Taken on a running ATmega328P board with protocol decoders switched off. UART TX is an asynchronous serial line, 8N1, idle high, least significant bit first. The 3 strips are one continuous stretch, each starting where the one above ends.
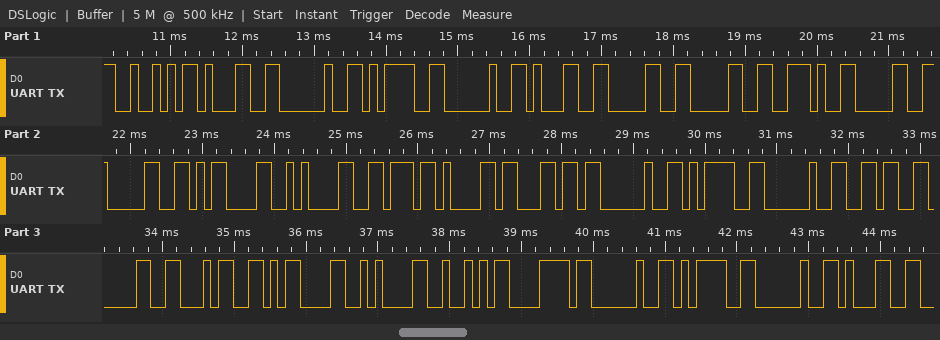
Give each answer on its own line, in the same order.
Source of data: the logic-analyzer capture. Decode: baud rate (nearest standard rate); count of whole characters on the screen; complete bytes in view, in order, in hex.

9600 baud
30
52 31 20 3D 20 31 30 30 2E 30 30 0D 0A 76 61 6C 20 3D 20 36 30 34 0D 0A 52 78 20 3D 20 31
